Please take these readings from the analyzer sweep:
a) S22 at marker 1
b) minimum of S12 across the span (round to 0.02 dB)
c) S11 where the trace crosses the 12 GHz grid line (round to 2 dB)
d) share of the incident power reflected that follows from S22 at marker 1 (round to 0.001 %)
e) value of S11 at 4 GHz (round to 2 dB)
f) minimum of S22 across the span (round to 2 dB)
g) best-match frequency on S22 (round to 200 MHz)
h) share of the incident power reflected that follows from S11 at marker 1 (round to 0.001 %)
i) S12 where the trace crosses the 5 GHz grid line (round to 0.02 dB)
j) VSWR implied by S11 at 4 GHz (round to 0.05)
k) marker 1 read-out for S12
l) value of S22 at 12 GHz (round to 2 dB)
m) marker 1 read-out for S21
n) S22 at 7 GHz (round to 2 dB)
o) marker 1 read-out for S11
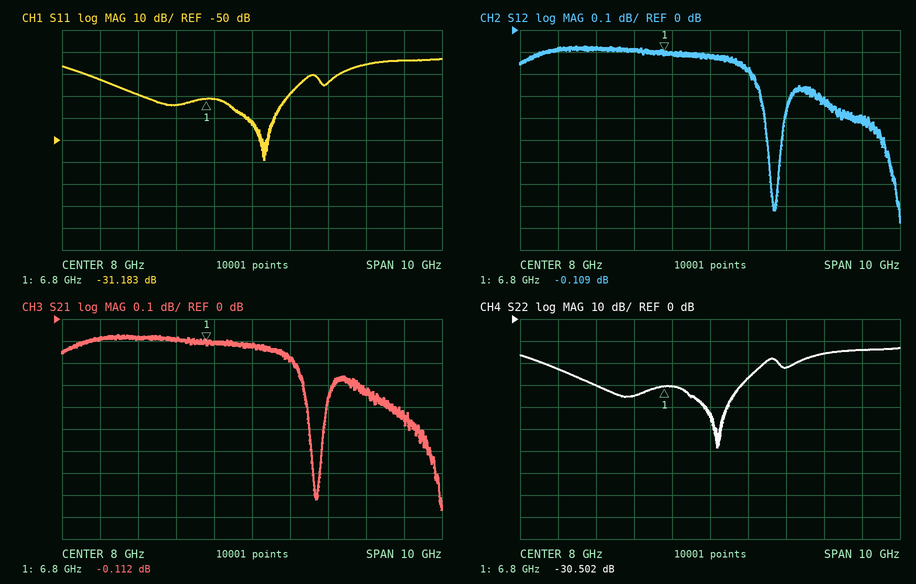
-30.502 dB
-0.88 dB
-14 dB
0.089 %
-22 dB
-58 dB
8.2 GHz
0.076 %
-0.08 dB
1.15
-0.109 dB
-14 dB
-0.112 dB
-30 dB
-31.183 dB
